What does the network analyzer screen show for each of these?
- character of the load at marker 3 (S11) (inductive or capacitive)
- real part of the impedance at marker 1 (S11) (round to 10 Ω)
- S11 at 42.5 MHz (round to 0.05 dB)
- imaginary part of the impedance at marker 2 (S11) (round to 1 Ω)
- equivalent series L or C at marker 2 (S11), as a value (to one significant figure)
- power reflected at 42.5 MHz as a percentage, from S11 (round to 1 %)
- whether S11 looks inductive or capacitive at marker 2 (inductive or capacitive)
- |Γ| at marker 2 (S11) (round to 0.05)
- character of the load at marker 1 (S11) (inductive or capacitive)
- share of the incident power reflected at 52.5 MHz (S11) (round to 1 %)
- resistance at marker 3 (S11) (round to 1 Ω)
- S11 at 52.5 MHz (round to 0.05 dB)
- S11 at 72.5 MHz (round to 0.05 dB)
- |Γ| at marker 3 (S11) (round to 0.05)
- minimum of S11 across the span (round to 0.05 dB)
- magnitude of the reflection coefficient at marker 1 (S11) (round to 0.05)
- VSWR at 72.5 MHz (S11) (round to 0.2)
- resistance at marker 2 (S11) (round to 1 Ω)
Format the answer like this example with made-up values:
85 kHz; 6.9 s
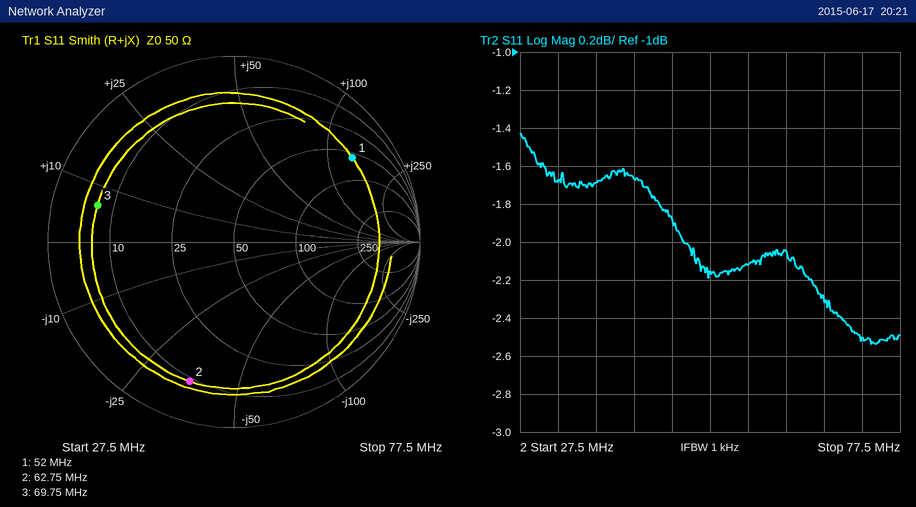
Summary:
inductive; 60 Ω; -1.65 dB; -36 Ω; 70 pF; 68 %; capacitive; 0.80; inductive; 61 %; 7 Ω; -2.15 dB; -2.50 dB; 0.75; -2.55 dB; 0.80; 7.0; 9 Ω
